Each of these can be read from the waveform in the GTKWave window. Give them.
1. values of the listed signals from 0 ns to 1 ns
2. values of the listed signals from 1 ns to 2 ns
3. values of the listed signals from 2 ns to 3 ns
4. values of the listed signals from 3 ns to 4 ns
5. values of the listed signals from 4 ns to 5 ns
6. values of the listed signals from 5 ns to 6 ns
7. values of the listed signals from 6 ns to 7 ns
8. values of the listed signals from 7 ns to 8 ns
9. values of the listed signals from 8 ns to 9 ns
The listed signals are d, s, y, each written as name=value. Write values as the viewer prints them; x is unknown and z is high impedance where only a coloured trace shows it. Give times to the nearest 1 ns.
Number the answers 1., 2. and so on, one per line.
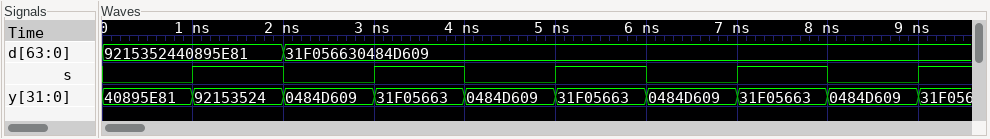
1. d=9215352440895E81, s=0, y=40895E81
2. d=9215352440895E81, s=1, y=92153524
3. d=31F056630484D609, s=0, y=0484D609
4. d=31F056630484D609, s=1, y=31F05663
5. d=31F056630484D609, s=0, y=0484D609
6. d=31F056630484D609, s=1, y=31F05663
7. d=31F056630484D609, s=0, y=0484D609
8. d=31F056630484D609, s=1, y=31F05663
9. d=31F056630484D609, s=0, y=0484D609
